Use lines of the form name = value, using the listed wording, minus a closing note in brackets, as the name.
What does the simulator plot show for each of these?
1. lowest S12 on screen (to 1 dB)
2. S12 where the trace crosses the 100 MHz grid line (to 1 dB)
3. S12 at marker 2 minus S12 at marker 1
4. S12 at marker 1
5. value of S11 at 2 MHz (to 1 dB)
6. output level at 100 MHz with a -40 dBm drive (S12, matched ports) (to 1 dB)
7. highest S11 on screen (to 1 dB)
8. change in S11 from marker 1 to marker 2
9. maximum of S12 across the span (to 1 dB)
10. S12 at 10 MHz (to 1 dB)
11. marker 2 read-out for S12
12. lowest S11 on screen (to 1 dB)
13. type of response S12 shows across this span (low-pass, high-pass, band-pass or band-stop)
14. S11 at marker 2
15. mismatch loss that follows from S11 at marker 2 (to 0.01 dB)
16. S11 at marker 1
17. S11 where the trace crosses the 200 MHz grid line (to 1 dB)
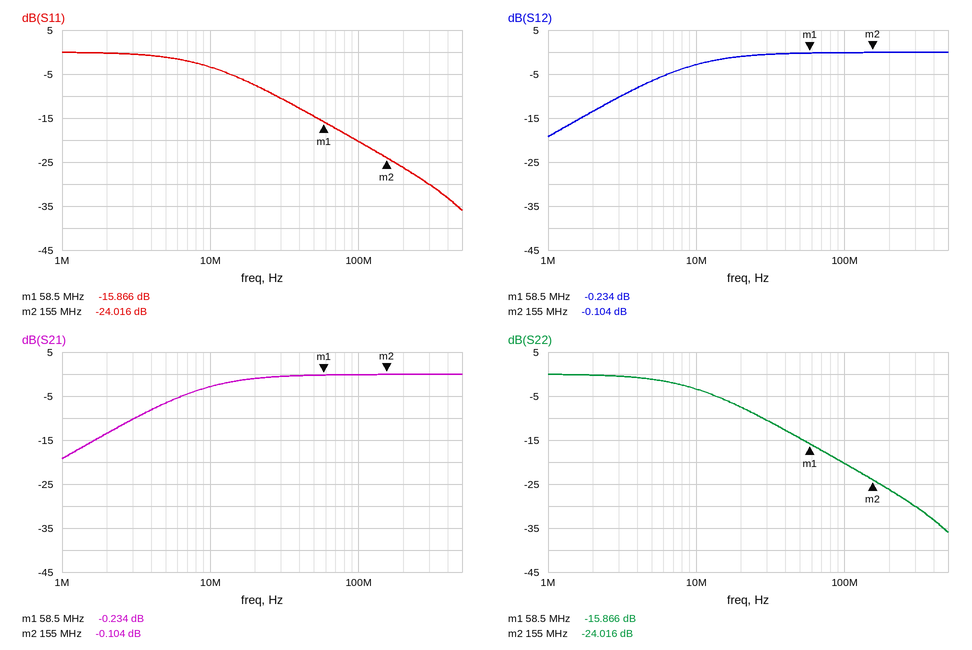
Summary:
lowest S12 on screen = -19 dB
S12 where the trace crosses the 100 MHz grid line = 0 dB
S12 at marker 2 minus S12 at marker 1 = 0.130 dB
S12 at marker 1 = -0.234 dB
value of S11 at 2 MHz = 0 dB
output level at 100 MHz with a -40 dBm drive (S12, matched ports) = -40 dBm
highest S11 on screen = 0 dB
change in S11 from marker 1 to marker 2 = -8.150 dB
maximum of S12 across the span = 0 dB
S12 at 10 MHz = -3 dB
marker 2 read-out for S12 = -0.104 dB
lowest S11 on screen = -36 dB
type of response S12 shows across this span = high-pass
S11 at marker 2 = -24.016 dB
mismatch loss that follows from S11 at marker 2 = 0.02 dB
S11 at marker 1 = -15.866 dB
S11 where the trace crosses the 200 MHz grid line = -26 dB
